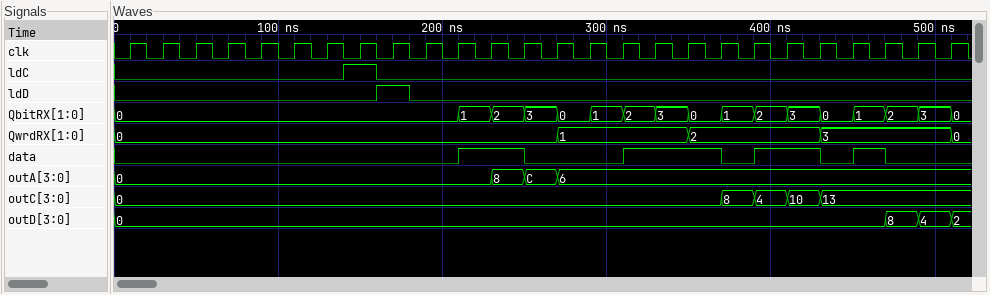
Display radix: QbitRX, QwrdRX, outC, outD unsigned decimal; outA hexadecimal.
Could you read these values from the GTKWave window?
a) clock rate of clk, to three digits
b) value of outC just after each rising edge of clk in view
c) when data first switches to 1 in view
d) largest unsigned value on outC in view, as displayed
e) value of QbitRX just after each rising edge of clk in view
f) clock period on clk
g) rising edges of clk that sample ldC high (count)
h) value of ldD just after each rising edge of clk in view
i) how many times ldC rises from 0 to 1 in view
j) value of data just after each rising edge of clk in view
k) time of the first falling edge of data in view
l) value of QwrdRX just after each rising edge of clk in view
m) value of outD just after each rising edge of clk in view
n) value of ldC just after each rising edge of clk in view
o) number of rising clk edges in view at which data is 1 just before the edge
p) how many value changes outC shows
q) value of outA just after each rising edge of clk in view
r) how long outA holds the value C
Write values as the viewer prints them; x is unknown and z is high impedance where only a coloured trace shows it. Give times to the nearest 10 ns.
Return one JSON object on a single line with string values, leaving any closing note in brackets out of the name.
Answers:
{"clock rate of clk, to three digits": "50.0 MHz", "value of outC just after each rising edge of clk in view": "0, 0, 0, 0, 0, 0, 0, 0, 0, 0, 0, 0, 0, 0, 0, 0, 0, 0, 8, 4, 10, 13, 13, 13, 13, 13", "when data first switches to 1 in view": "210 ns", "largest unsigned value on outC in view, as displayed": "13", "value of QbitRX just after each rising edge of clk in view": "0, 0, 0, 0, 0, 0, 0, 0, 0, 0, 1, 2, 3, 0, 1, 2, 3, 0, 1, 2, 3, 0, 1, 2, 3, 0", "clock period on clk": "20 ns", "rising edges of clk that sample ldC high": "1", "value of ldD just after each rising edge of clk in view": "0 0 0 0 0 0 0 0 1 0 0 0 0 0 0 0 0 0 0 0 0 0 0 0 0 0", "how many times ldC rises from 0 to 1 in view": "1", "value of data just after each rising edge of clk in view": "0 0 0 0 0 0 0 0 0 0 1 1 0 0 0 1 1 1 0 1 1 0 1 0 0 0", "time of the first falling edge of data in view": "250 ns", "value of QwrdRX just after each rising edge of clk in view": "0, 0, 0, 0, 0, 0, 0, 0, 0, 0, 0, 0, 0, 1, 1, 1, 1, 2, 2, 2, 2, 3, 3, 3, 3, 0", "value of outD just after each rising edge of clk in view": "0, 0, 0, 0, 0, 0, 0, 0, 0, 0, 0, 0, 0, 0, 0, 0, 0, 0, 0, 0, 0, 0, 0, 8, 4, 2", "value of ldC just after each rising edge of clk in view": "0 0 0 0 0 0 0 1 0 0 0 0 0 0 0 0 0 0 0 0 0 0 0 0 0 0", "number of rising clk edges in view at which data is 1 just before the edge": "8", "how many value changes outC shows": "4", "value of outA just after each rising edge of clk in view": "0, 0, 0, 0, 0, 0, 0, 0, 0, 0, 0, 8, C, 6, 6, 6, 6, 6, 6, 6, 6, 6, 6, 6, 6, 6", "how long outA holds the value C": "20 ns"}
